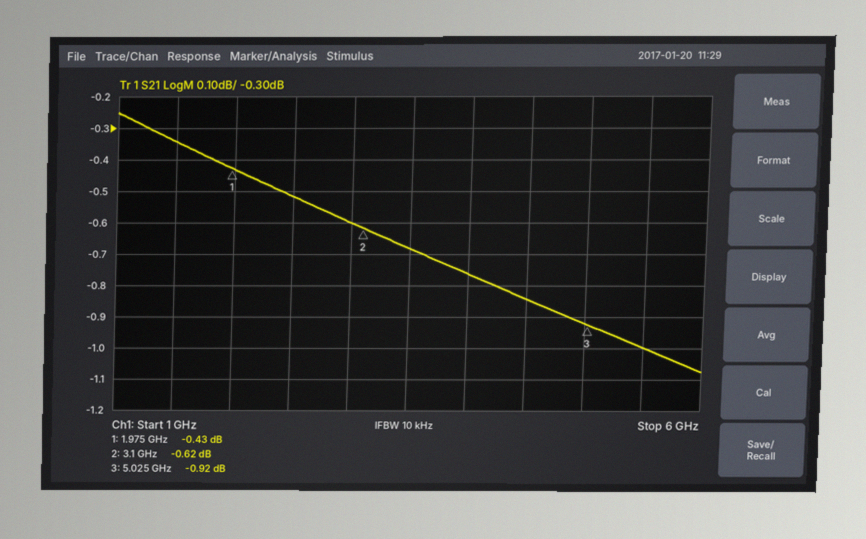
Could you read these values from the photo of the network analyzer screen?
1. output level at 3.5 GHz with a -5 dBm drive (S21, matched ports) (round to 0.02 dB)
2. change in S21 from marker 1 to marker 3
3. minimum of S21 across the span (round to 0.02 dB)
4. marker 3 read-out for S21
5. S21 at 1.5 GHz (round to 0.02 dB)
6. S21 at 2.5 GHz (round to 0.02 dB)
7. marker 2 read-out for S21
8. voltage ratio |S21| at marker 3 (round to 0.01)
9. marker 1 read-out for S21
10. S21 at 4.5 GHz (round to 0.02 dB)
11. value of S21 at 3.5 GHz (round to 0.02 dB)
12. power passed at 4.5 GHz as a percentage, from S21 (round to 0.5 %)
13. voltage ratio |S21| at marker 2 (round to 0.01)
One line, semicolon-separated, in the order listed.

-5.68 dBm; -0.49 dB; -1.08 dB; -0.92 dB; -0.34 dB; -0.52 dB; -0.62 dB; 0.90; -0.43 dB; -0.84 dB; -0.68 dB; 82.5 %; 0.93
